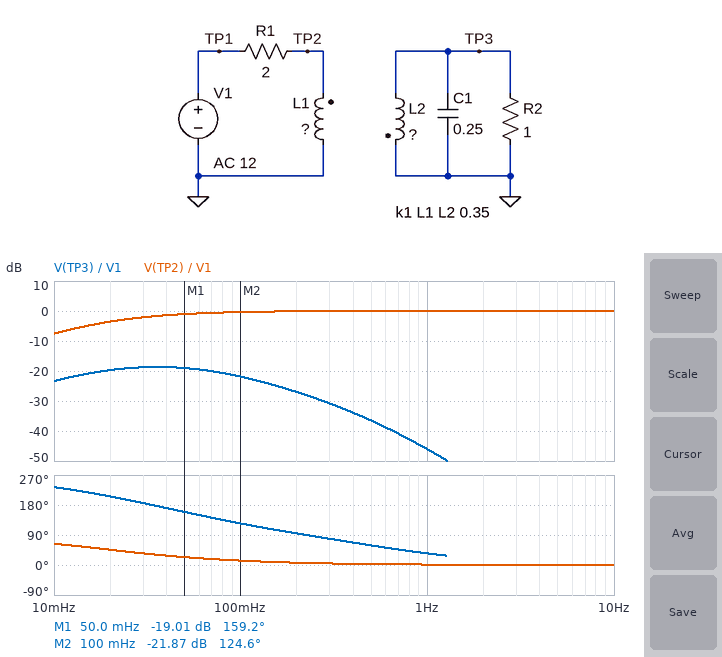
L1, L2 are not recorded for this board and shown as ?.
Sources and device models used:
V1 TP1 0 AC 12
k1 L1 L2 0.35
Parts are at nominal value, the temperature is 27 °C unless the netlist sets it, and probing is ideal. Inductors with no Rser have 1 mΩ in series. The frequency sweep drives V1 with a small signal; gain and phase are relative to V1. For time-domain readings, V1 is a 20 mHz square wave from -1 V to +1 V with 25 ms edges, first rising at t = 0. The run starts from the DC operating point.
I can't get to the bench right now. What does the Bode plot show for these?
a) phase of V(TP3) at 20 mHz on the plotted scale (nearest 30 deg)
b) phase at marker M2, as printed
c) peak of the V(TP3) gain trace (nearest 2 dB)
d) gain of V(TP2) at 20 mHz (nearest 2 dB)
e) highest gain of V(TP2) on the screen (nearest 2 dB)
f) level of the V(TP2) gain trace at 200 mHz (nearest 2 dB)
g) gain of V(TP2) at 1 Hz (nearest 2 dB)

210 deg
124.6 deg
-18 dB
-4 dB
0 dB
0 dB
0 dB
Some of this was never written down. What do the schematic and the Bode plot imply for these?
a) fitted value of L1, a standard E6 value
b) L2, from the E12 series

15 H
3.3 H
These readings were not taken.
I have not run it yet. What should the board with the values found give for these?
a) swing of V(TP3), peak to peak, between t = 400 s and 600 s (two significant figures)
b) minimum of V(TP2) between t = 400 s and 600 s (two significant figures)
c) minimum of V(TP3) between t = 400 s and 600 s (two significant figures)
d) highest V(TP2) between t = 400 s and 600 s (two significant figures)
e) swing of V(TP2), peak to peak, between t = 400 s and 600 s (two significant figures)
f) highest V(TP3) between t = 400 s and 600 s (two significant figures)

340 mV
-1.9 V
-170 mV
1.9 V
3.8 V
170 mV
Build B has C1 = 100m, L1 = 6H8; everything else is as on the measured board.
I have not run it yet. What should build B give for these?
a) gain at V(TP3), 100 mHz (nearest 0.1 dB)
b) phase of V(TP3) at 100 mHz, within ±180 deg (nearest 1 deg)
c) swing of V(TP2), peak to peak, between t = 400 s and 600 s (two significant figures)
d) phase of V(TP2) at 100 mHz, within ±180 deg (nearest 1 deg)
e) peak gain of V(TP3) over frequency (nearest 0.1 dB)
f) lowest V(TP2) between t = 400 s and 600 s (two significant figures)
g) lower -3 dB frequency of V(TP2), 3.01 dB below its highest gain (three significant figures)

-19.6 dB
143 deg
4.0 V
27 deg
-18.0 dB
-2.0 V
53.6 mHz
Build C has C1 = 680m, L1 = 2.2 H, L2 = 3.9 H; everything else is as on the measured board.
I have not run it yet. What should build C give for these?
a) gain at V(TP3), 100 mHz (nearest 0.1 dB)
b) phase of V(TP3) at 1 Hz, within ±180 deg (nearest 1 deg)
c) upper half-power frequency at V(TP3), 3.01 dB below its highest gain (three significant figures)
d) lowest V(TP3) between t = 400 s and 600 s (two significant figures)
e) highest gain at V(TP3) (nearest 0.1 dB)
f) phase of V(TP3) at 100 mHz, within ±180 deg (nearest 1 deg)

-19.2 dB
23 deg
174 mHz
-170 mV
-18.9 dB
149 deg
